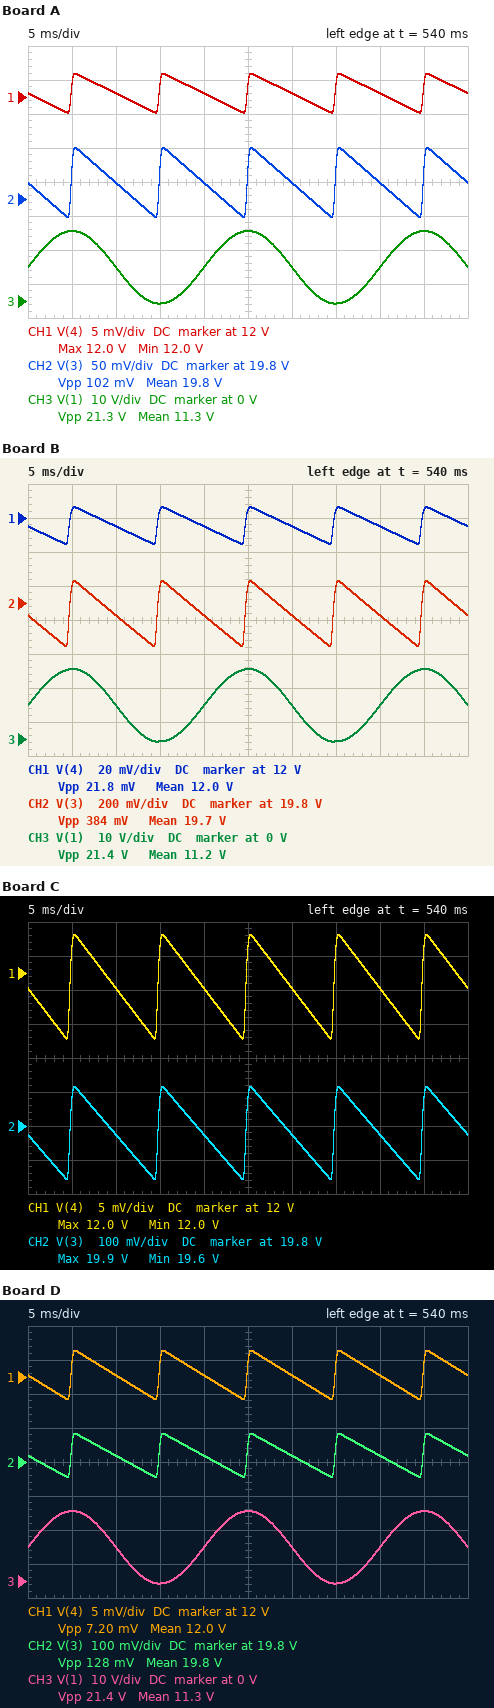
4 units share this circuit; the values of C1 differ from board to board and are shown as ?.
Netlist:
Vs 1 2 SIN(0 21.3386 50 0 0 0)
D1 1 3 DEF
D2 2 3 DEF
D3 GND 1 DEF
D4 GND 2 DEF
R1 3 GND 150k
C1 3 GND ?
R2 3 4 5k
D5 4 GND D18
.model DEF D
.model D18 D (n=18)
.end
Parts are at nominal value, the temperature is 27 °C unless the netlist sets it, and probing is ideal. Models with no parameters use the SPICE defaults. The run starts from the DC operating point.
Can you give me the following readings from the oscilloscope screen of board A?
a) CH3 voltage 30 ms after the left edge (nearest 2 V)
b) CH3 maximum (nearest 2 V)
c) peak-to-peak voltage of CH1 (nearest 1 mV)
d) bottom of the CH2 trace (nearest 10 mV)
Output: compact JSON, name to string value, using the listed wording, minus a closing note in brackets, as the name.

{"CH3 voltage 30 ms after the left edge": "10 V", "CH3 maximum": "20 V", "peak-to-peak voltage of CH1": "6 mV", "bottom of the CH2 trace": "19.77 V"}
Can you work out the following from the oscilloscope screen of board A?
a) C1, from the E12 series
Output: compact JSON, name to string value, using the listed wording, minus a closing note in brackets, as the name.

{"C1, from the E12 series": "150 µF"}
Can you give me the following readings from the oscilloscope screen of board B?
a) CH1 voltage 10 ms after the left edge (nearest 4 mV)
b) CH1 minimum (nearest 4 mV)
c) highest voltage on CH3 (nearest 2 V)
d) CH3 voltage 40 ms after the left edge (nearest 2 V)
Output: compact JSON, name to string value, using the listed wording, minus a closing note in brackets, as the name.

{"CH1 voltage 10 ms after the left edge": "11.996 V", "CH1 minimum": "11.984 V", "highest voltage on CH3": "20 V", "CH3 voltage 40 ms after the left edge": "10 V"}
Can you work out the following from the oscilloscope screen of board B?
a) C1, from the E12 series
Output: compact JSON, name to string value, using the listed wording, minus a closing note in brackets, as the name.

{"C1, from the E12 series": "39 µF"}
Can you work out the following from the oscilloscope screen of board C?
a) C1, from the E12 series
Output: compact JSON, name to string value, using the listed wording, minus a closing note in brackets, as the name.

{"C1, from the E12 series": "56 µF"}
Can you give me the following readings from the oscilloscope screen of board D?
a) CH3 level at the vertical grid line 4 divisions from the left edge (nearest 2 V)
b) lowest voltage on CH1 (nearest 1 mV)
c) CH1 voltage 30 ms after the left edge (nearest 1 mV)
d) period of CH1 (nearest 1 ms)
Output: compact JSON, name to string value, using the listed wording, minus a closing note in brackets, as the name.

{"CH3 level at the vertical grid line 4 divisions from the left edge": "10 V", "lowest voltage on CH1": "11.997 V", "CH1 voltage 30 ms after the left edge": "12.000 V", "period of CH1": "10 ms"}
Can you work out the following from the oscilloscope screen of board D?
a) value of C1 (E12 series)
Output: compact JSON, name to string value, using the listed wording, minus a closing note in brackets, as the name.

{"value of C1": "120 µF"}
